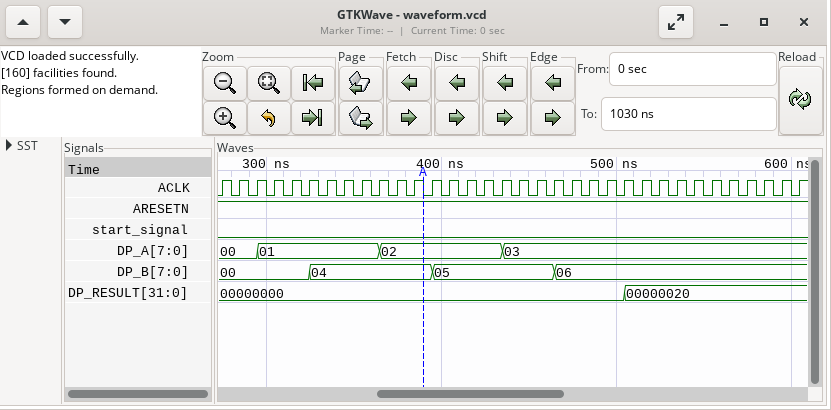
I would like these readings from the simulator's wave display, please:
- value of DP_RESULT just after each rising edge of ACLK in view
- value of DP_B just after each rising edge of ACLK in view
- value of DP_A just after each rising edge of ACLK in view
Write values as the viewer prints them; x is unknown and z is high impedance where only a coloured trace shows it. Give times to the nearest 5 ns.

00000000, 00000000, 00000000, 00000000, 00000000, 00000000, 00000000, 00000000, 00000000, 00000000, 00000000, 00000000, 00000000, 00000000, 00000000, 00000000, 00000000, 00000000, 00000000, 00000000, 00000000, 00000000, 00000000, 00000020, 00000020, 00000020, 00000020, 00000020, 00000020, 00000020, 00000020, 00000020, 00000020, 00000020
00, 00, 00, 00, 00, 04, 04, 04, 04, 04, 04, 04, 05, 05, 05, 05, 05, 05, 05, 06, 06, 06, 06, 06, 06, 06, 06, 06, 06, 06, 06, 06, 06, 06
00, 00, 01, 01, 01, 01, 01, 01, 01, 02, 02, 02, 02, 02, 02, 02, 03, 03, 03, 03, 03, 03, 03, 03, 03, 03, 03, 03, 03, 03, 03, 03, 03, 03
